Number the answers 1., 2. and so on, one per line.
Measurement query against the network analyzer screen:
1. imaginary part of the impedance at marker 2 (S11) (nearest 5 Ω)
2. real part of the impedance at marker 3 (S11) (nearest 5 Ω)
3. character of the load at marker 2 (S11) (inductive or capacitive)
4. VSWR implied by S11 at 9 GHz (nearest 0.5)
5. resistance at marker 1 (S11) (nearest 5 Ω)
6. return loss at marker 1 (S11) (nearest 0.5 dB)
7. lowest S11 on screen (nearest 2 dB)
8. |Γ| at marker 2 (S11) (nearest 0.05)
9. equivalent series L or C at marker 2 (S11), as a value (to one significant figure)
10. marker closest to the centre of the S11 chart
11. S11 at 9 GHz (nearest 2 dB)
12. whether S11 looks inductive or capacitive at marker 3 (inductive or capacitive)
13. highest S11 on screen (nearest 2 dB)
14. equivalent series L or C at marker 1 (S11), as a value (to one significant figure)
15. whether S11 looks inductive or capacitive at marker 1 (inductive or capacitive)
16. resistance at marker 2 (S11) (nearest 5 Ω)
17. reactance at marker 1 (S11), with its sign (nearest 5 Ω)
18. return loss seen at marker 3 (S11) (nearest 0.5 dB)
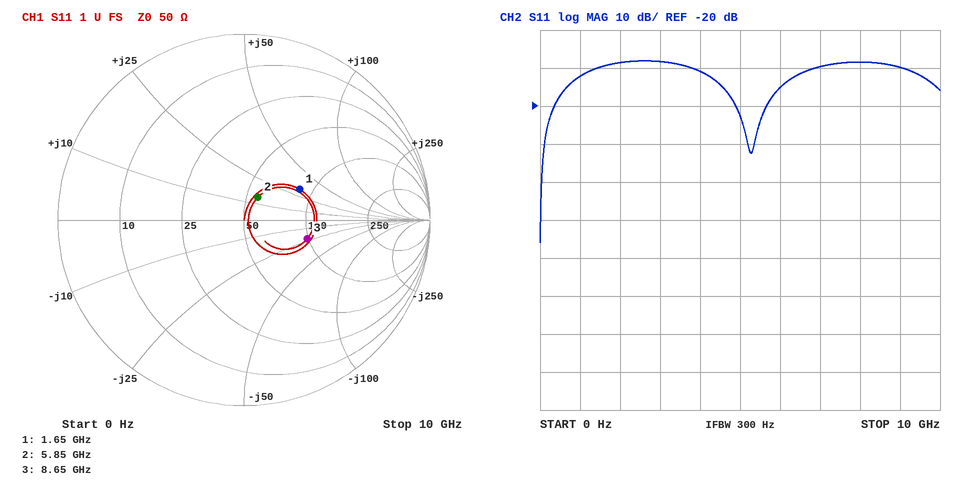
1. +15 Ω
2. 100 Ω
3. inductive
4. 2.0
5. 85 Ω
6. 9.5 dB
7. -56 dB
8. 0.15
9. 400 pH
10. marker 2
11. -10 dB
12. capacitive
13. -8 dB
14. 3 nH
15. inductive
16. 55 Ω
17. +30 Ω
18. 9.0 dB
